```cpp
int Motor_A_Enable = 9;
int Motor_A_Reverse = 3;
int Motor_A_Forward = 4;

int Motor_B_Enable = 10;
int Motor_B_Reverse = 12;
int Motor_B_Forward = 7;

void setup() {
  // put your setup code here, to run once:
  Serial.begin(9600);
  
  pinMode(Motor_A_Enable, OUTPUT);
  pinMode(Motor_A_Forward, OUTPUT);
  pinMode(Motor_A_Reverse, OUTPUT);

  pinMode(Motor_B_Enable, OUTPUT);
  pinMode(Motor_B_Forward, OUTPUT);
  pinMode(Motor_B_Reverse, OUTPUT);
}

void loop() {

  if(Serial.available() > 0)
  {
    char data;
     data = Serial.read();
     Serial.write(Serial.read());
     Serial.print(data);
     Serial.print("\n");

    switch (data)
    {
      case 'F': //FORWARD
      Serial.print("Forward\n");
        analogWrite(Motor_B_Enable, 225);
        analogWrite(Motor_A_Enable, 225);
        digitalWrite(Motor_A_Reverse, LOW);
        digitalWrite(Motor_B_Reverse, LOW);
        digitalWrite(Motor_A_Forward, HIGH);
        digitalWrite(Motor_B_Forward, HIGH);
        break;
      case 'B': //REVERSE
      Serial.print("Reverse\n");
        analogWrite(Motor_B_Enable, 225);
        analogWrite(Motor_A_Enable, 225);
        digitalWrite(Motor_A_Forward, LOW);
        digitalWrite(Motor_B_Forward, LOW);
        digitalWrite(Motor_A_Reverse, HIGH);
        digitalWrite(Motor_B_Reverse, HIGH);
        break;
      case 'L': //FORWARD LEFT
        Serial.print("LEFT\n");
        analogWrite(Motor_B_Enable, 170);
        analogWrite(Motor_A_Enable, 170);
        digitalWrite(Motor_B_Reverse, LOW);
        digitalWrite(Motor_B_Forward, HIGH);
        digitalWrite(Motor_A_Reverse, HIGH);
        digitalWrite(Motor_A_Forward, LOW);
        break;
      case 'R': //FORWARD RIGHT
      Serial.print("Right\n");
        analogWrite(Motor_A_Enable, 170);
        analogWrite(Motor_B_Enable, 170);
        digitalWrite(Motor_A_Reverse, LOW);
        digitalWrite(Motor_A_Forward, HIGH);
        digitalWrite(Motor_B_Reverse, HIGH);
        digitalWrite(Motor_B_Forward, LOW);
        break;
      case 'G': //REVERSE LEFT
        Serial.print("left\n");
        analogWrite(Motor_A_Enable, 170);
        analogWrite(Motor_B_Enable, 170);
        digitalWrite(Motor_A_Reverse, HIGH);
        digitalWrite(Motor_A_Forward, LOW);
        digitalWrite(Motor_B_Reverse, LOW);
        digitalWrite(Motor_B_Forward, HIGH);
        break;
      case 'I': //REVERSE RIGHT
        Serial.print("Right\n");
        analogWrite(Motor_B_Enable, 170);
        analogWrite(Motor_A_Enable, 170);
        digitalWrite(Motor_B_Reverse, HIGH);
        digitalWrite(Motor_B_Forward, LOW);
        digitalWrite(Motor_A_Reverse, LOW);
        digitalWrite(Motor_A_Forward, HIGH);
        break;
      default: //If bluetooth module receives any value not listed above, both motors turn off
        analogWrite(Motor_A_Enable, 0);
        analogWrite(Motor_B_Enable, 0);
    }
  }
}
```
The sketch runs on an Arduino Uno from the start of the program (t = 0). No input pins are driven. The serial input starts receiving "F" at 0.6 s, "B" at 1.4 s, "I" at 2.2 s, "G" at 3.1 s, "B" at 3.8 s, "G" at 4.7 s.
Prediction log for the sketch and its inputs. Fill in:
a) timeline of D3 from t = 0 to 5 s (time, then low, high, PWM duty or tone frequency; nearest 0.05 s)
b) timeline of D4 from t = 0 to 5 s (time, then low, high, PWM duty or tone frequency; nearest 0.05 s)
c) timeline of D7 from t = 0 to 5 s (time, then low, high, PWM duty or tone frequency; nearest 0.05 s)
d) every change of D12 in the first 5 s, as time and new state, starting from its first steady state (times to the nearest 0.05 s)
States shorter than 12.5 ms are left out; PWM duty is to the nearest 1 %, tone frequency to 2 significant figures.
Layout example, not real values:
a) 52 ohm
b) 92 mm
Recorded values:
a) 0 s low; 1.4 s high; 2.2 s low; 3.1 s high
b) 0 s low; 0.6 s high; 1.4 s low; 2.2 s high; 3.1 s low
c) 0 s low; 0.6 s high; 1.4 s low; 3.1 s high; 3.8 s low; 4.7 s high
d) 0 s low; 1.4 s high; 3.1 s low; 3.8 s high; 4.7 s low
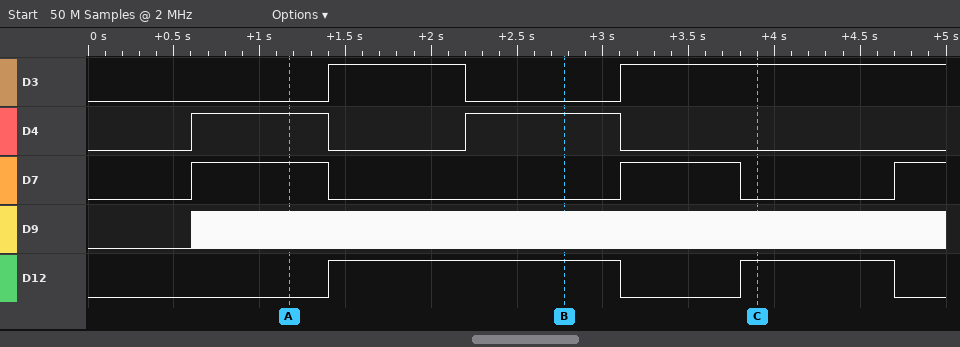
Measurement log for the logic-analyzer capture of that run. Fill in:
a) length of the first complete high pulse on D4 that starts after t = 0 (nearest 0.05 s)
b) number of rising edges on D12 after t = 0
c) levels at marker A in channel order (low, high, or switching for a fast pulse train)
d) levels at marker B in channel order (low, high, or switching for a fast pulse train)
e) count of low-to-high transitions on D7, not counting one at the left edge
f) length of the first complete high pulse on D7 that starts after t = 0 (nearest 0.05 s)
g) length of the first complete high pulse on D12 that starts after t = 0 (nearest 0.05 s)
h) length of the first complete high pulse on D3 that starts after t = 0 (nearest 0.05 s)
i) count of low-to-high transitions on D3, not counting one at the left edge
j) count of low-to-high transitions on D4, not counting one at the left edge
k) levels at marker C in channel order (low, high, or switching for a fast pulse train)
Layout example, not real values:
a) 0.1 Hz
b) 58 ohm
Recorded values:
a) 0.80 s
b) 2
c) D3 low, D4 high, D7 high, D9 switching, D12 low
d) D3 low, D4 high, D7 low, D9 switching, D12 high
e) 3
f) 0.80 s
g) 1.70 s
h) 0.80 s
i) 2
j) 2
k) D3 high, D4 low, D7 low, D9 switching, D12 high
